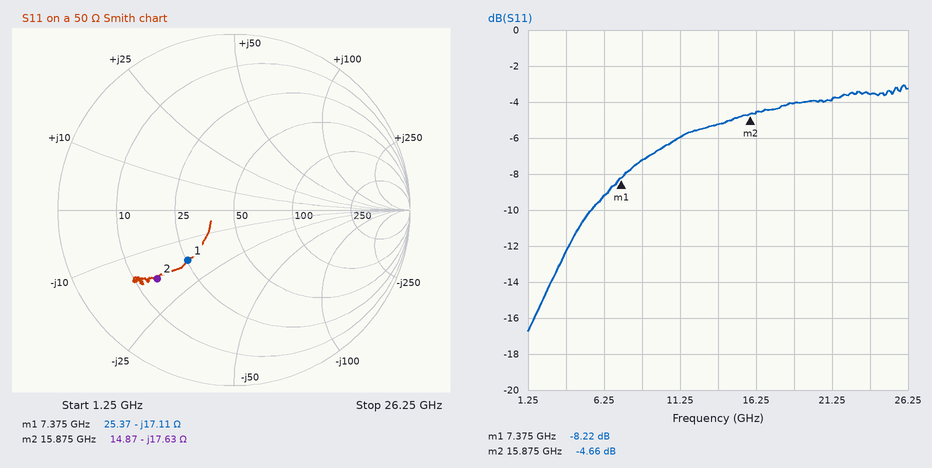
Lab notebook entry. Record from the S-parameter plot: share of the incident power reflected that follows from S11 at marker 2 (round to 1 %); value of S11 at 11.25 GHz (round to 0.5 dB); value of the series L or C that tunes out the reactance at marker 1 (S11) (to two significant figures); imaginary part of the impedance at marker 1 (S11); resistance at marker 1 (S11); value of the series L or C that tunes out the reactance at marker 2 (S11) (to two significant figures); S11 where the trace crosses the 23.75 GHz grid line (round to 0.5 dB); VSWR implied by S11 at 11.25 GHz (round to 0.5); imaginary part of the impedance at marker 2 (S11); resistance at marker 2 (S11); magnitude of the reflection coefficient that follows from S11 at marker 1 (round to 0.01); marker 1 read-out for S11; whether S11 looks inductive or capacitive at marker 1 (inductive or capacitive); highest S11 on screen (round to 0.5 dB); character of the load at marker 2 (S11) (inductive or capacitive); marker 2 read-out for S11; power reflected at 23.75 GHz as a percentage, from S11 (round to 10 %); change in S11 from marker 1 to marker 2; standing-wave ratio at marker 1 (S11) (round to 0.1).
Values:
34 %
-6.0 dB
370 pH
-17.11 Ω
25.37 Ω
180 pH
-3.5 dB
3.0
-17.63 Ω
14.87 Ω
0.39
-8.22 dB
capacitive
-3.0 dB
capacitive
-4.66 dB
40 %
3.56 dB
2.3
